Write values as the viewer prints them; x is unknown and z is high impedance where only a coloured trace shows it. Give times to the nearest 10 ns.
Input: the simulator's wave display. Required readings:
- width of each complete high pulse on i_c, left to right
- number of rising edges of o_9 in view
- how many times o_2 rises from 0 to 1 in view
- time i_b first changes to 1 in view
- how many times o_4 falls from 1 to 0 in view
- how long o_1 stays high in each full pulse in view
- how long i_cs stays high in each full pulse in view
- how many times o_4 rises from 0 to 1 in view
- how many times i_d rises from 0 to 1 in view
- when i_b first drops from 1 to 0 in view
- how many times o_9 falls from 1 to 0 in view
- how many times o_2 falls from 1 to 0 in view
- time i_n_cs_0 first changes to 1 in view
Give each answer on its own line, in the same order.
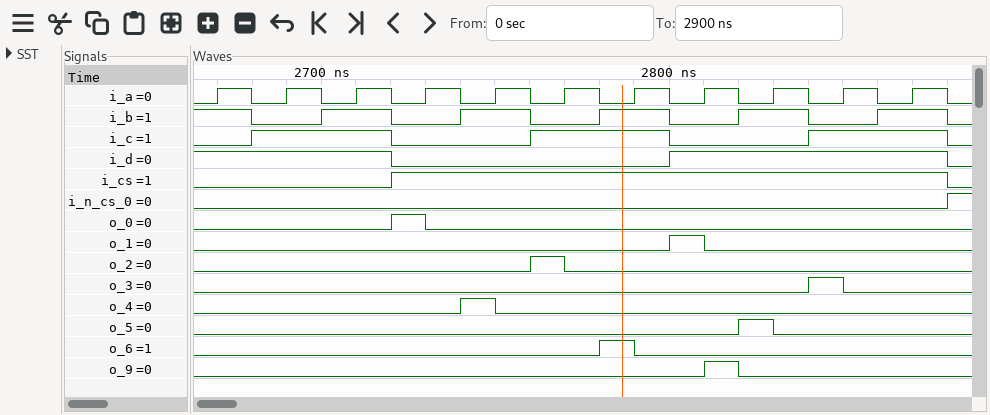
40 ns, 40 ns, 40 ns
1
1
2700 ns
1
10 ns
160 ns
1
1
2680 ns
1
1
2880 ns
